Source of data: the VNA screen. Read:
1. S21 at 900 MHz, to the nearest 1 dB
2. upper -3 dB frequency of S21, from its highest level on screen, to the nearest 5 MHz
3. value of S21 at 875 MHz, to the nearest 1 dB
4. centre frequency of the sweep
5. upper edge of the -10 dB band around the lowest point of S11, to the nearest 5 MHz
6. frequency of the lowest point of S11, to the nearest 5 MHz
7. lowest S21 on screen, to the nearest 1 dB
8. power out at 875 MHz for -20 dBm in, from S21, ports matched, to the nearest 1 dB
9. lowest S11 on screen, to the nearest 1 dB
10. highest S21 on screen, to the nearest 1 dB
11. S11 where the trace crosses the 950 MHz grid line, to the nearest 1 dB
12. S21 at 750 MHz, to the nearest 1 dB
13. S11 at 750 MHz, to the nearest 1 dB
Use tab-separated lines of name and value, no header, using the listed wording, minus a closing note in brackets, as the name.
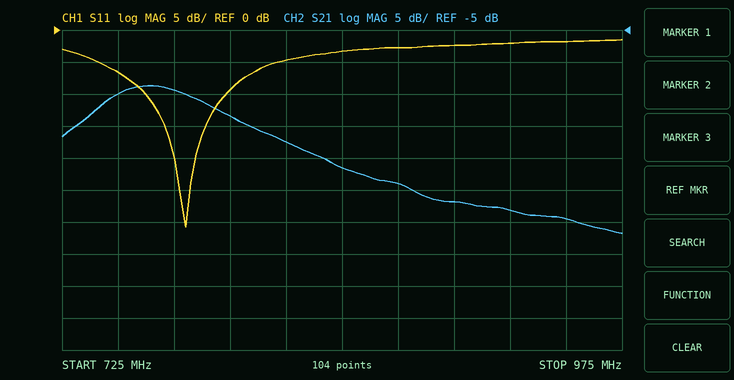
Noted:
S21 at 900 MHz, to the nearest 1 dB	-32 dB
upper -3 dB frequency of S21, from its highest level on screen, to the nearest 5 MHz	790 MHz
value of S21 at 875 MHz, to the nearest 1 dB	-29 dB
centre frequency of the sweep	850 MHz
upper edge of the -10 dB band around the lowest point of S11, to the nearest 5 MHz	800 MHz
frequency of the lowest point of S11, to the nearest 5 MHz	780 MHz
lowest S21 on screen, to the nearest 1 dB	-37 dB
power out at 875 MHz for -20 dBm in, from S21, ports matched, to the nearest 1 dB	-49 dBm
lowest S11 on screen, to the nearest 1 dB	-31 dB
highest S21 on screen, to the nearest 1 dB	-14 dB
S11 where the trace crosses the 950 MHz grid line, to the nearest 1 dB	-2 dB
S21 at 750 MHz, to the nearest 1 dB	-15 dB
S11 at 750 MHz, to the nearest 1 dB	-7 dB
